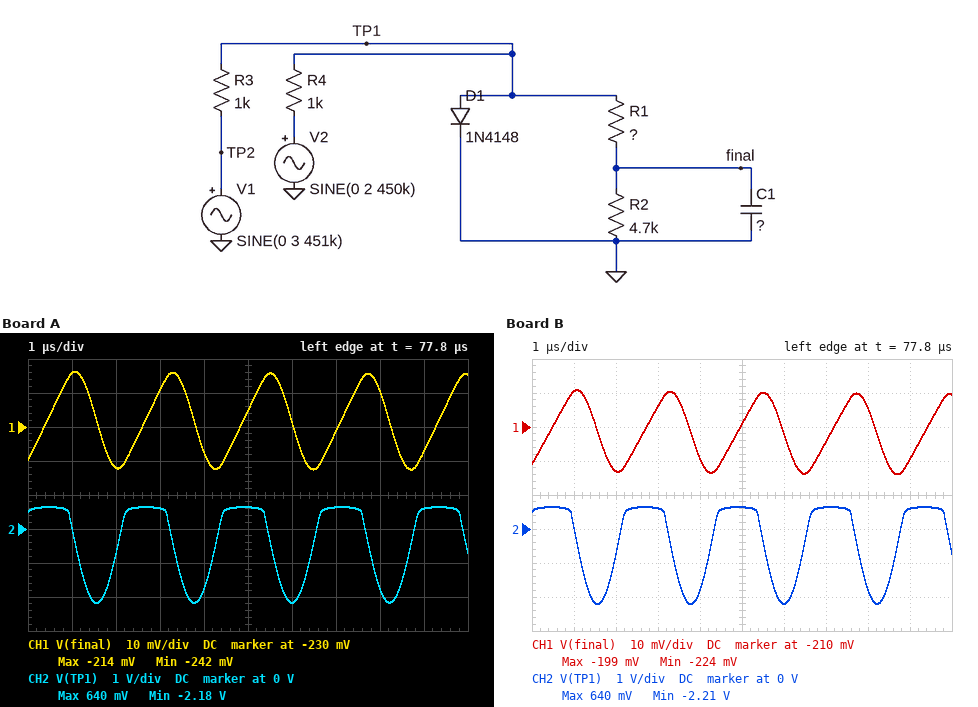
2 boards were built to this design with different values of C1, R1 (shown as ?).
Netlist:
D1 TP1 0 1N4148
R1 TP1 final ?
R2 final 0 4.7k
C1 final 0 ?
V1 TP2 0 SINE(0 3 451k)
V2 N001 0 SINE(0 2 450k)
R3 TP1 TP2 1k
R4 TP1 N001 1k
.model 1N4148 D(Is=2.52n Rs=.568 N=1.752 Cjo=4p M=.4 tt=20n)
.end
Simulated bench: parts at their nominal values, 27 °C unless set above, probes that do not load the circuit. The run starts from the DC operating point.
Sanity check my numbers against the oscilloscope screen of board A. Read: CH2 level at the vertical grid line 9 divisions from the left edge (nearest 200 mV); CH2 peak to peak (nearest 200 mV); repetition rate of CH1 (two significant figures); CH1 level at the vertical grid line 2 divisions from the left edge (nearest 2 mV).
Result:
600 mV
2.8 V
450 kHz
-242 mV
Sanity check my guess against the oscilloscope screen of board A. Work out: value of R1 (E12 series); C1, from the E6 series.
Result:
3.9 kΩ
10 nF
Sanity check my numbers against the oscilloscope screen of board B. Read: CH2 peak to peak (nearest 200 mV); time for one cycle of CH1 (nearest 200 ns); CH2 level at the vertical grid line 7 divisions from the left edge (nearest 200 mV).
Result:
2.8 V
2.2 µs
600 mV
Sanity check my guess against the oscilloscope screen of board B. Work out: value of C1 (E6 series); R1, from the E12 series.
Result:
10 nF
4.7 kΩ
